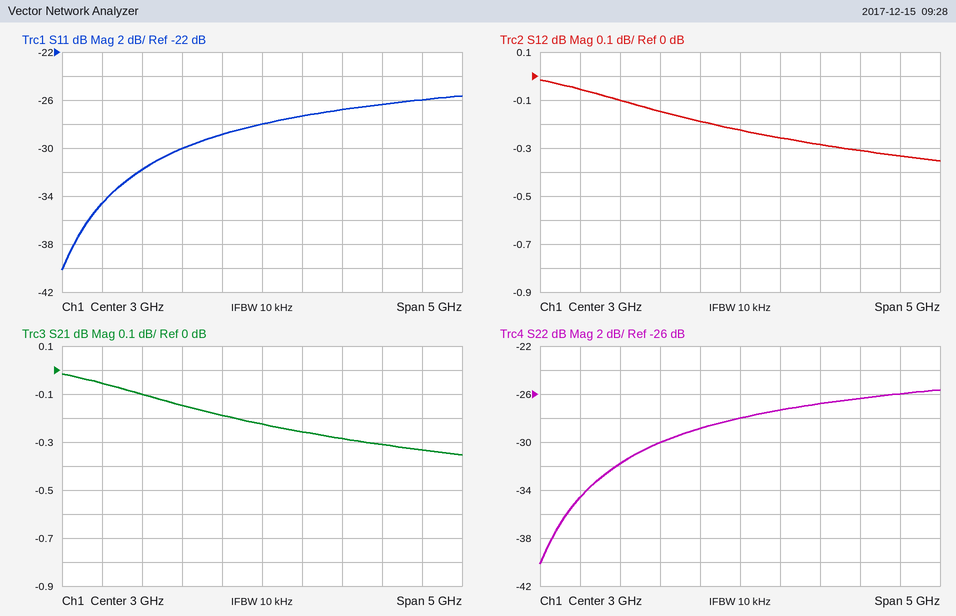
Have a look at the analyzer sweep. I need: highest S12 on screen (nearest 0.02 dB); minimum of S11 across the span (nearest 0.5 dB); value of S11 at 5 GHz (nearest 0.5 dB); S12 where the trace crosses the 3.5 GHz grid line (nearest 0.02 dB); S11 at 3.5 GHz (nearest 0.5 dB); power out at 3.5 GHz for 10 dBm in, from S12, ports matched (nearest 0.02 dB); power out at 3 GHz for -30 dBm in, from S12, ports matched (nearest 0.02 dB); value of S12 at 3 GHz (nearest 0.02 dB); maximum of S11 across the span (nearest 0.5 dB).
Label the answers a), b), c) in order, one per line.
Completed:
a) -0.02 dB
b) -40.0 dB
c) -26.0 dB
d) -0.26 dB
e) -27.5 dB
f) 9.74 dBm
g) -30.22 dBm
h) -0.22 dB
i) -25.5 dB
